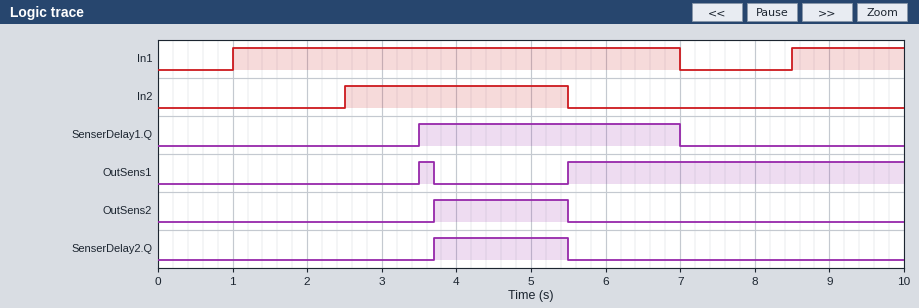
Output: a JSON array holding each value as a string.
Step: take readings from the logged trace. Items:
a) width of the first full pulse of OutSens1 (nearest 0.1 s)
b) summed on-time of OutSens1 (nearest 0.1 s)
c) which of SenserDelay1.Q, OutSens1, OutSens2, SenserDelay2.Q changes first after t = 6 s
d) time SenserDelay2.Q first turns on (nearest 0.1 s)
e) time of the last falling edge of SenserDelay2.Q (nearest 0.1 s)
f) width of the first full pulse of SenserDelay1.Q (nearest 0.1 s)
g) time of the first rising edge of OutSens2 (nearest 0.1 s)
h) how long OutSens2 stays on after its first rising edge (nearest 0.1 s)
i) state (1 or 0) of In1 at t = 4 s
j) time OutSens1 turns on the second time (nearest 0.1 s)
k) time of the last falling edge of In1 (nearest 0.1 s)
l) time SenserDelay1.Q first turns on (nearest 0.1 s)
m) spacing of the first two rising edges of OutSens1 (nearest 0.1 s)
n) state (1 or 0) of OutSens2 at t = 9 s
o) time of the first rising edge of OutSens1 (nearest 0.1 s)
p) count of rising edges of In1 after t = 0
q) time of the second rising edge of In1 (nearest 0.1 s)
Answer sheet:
["0.2 s", "4.7 s", "SenserDelay1.Q", "3.7 s", "5.5 s", "3.5 s", "3.7 s", "1.8 s", "1", "5.5 s", "7.0 s", "3.5 s", "2.0 s", "0", "3.5 s", "2", "8.5 s"]
